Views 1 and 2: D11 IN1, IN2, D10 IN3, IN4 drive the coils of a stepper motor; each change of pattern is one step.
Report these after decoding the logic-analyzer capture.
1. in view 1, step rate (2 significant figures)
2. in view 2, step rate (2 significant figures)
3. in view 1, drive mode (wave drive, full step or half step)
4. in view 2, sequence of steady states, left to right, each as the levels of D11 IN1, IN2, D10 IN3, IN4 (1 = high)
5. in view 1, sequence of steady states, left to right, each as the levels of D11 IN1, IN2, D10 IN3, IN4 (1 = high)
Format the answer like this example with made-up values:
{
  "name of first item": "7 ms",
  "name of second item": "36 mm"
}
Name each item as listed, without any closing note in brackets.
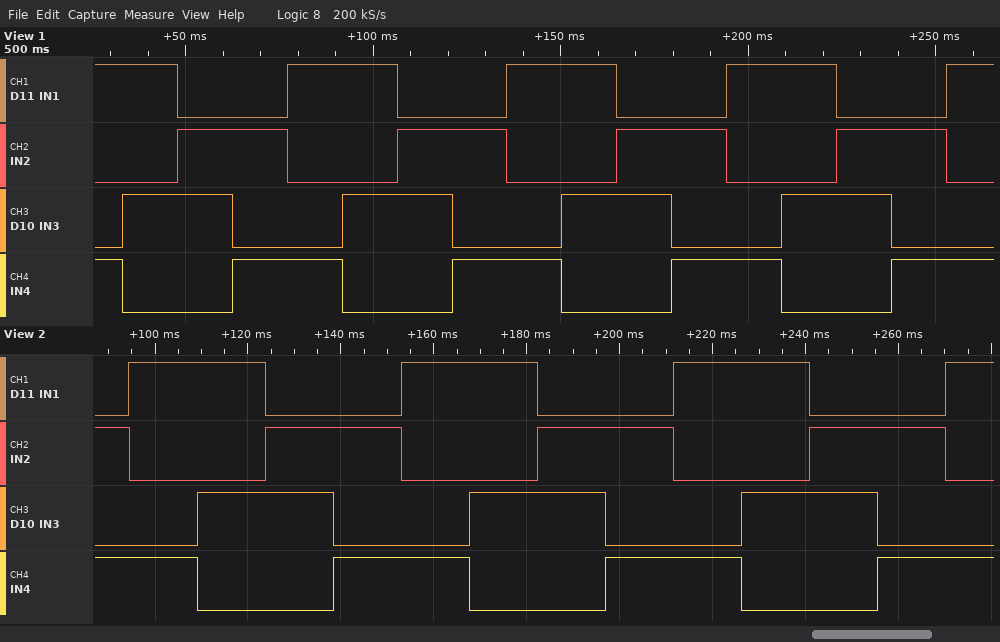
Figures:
{
  "in view 1, step rate": "68 steps/s",
  "in view 2, step rate": "68 steps/s",
  "in view 1, drive mode": "full step",
  "in view 2, sequence of steady states, left to right, each as the levels of D11 IN1, IN2, D10 IN3, IN4": "0101 1001 1010 0110 0101 1001 1010 0110 0101 1001 1010 0110 0101 1001",
  "in view 1, sequence of steady states, left to right, each as the levels of D11 IN1, IN2, D10 IN3, IN4": "1001 1010 0110 0101 1001 1010 0110 0101 1001 1010 0110 0101 1001 1010 0110 0101 1001"
}
